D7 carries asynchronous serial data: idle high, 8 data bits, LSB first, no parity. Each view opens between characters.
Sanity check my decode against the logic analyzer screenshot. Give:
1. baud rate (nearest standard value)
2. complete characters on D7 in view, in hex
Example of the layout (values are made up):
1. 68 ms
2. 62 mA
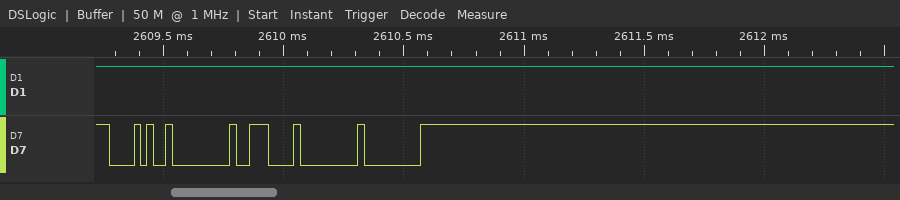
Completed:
1. 38400 baud
2. 28, 00, 0E, 00, 00
